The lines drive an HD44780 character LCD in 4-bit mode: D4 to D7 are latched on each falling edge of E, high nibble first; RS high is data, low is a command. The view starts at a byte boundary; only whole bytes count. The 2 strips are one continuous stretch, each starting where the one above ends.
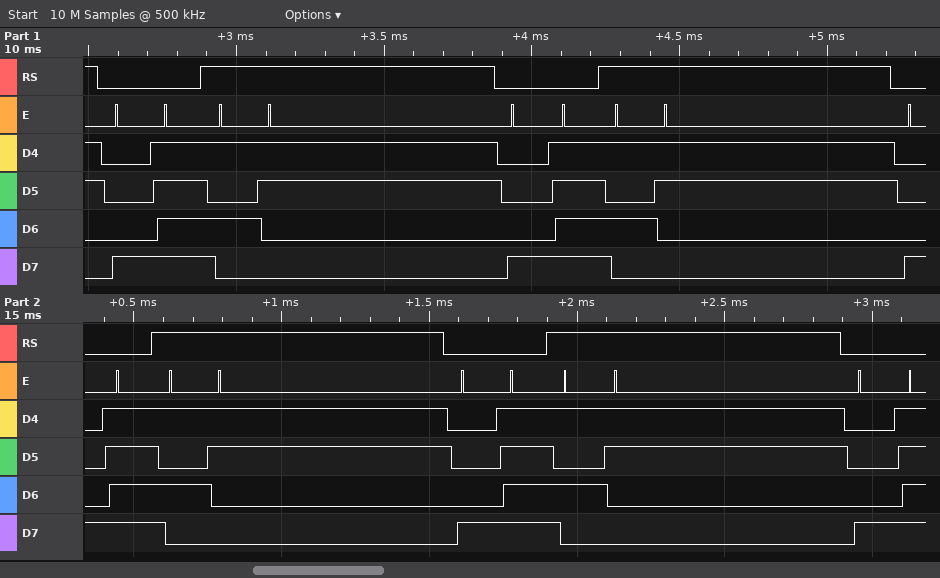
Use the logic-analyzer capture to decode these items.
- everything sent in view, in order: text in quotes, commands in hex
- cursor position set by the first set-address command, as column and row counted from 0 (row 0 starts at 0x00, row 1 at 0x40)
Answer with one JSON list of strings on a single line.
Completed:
["0x8F \"S\" 0x8F \"S\" 0x8F \"S\" 0x8F \"S\" 0x8F", "column 15, row 0"]
